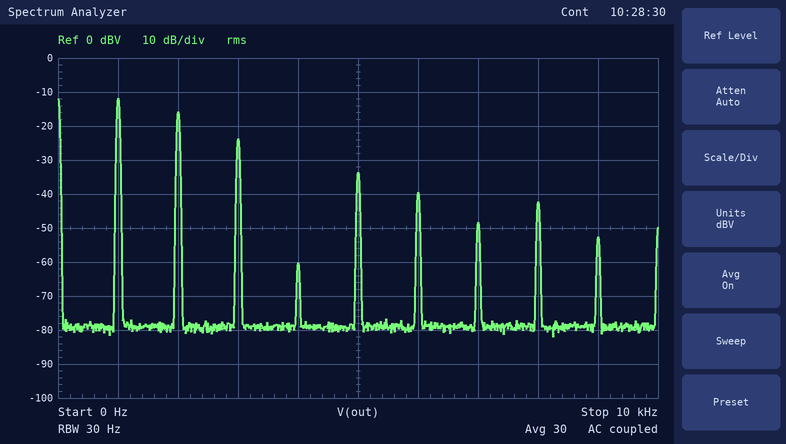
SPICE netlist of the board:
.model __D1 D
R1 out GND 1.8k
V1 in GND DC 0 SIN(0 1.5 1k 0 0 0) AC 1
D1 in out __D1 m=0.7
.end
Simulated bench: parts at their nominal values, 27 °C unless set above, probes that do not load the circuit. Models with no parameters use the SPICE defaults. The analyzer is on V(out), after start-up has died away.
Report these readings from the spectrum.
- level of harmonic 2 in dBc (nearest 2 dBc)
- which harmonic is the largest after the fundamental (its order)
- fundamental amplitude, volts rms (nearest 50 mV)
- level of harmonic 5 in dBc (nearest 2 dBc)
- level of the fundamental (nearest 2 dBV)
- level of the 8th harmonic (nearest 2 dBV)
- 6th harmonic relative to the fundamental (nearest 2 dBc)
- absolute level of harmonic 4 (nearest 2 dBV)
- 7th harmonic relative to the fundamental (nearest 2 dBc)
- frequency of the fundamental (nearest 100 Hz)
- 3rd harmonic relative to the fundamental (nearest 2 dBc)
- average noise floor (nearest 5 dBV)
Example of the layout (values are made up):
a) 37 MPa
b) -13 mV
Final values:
a) -4 dBc
b) 2
c) 250 mV
d) -22 dBc
e) -12 dBV
f) -42 dBV
g) -28 dBc
h) -60 dBV
i) -36 dBc
j) 1.0 kHz
k) -12 dBc
l) -80 dBV
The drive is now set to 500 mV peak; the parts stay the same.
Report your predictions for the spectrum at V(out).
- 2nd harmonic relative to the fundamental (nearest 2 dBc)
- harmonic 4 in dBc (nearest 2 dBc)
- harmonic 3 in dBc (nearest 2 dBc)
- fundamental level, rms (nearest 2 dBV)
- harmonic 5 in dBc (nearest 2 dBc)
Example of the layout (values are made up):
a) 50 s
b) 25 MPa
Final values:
a) 0 dBc
b) -4 dBc
c) -2 dBc
d) -68 dBV
e) -6 dBc
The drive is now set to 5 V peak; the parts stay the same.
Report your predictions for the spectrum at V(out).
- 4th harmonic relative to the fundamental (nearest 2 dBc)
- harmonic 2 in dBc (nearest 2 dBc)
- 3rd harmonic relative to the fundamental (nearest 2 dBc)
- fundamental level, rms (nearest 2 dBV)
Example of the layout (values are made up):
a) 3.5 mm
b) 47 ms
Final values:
a) -22 dBc
b) -6 dBc
c) -24 dBc
d) 4 dBV
